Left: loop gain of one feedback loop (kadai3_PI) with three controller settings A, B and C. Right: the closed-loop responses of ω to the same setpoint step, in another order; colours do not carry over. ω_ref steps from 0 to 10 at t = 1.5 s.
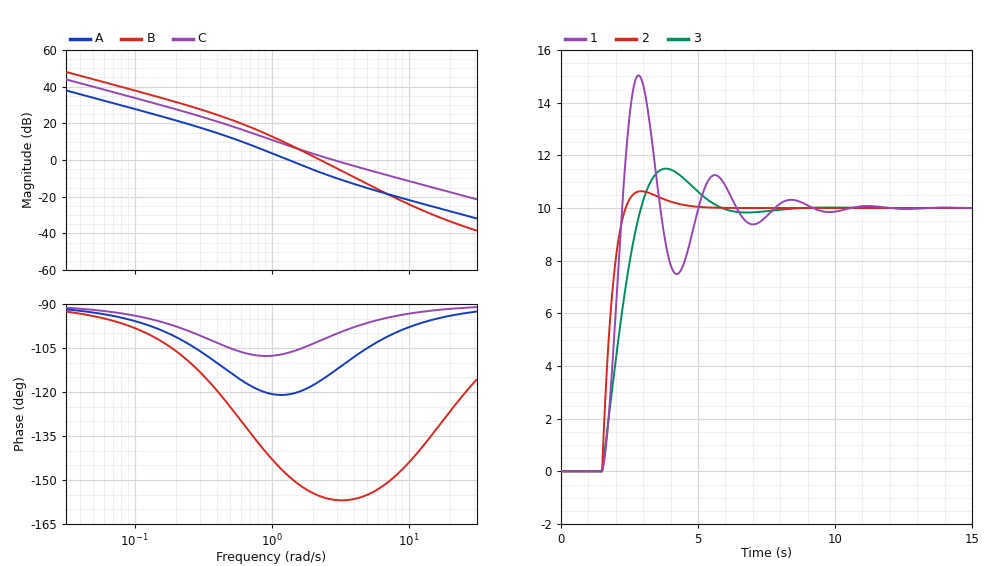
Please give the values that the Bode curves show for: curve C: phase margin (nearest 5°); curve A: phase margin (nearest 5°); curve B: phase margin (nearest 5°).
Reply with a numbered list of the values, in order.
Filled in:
1. 80°
2. 60°
3. 25°
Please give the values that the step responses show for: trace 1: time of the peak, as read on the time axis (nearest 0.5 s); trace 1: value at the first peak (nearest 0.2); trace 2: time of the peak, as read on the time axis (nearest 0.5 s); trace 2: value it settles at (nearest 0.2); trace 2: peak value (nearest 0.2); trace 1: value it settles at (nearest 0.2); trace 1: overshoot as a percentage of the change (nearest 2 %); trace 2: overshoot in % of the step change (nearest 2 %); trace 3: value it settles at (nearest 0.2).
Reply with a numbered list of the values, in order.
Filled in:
1. 3.0 s
2. 15.0
3. 3.0 s
4. 10.0
5. 10.6
6. 10.0
7. 50 %
8. 6 %
9. 10.0
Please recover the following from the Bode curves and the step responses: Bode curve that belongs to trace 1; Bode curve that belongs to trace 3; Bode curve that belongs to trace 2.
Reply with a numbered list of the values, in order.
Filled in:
1. B
2. A
3. C
